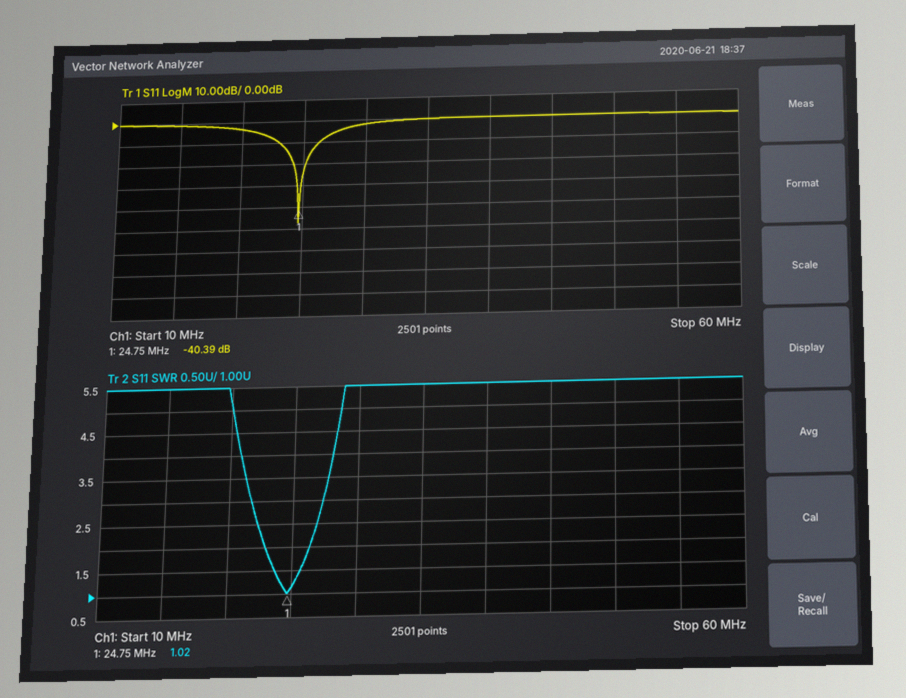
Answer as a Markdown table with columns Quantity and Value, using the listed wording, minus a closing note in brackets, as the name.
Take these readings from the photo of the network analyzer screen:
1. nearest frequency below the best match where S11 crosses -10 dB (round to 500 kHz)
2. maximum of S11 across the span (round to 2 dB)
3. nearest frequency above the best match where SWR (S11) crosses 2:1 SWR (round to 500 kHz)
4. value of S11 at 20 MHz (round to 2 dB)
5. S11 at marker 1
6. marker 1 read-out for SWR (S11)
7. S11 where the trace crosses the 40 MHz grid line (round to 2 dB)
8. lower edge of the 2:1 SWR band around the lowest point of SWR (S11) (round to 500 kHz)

| Quantity | Value |
|---|---|
| nearest frequency below the best match where S11 crosses -10 dB | 23.0 MHz |
| maximum of S11 across the span | 0 dB |
| nearest frequency above the best match where SWR (S11) crosses 2:1 SWR | 26.5 MHz |
| value of S11 at 20 MHz | -4 dB |
| S11 at marker 1 | -40.39 dB |
| marker 1 read-out for SWR | 1.02 |
| S11 where the trace crosses the 40 MHz grid line | 0 dB |
| lower edge of the 2:1 SWR band around the lowest point of SWR (S11) | 23.0 MHz |
